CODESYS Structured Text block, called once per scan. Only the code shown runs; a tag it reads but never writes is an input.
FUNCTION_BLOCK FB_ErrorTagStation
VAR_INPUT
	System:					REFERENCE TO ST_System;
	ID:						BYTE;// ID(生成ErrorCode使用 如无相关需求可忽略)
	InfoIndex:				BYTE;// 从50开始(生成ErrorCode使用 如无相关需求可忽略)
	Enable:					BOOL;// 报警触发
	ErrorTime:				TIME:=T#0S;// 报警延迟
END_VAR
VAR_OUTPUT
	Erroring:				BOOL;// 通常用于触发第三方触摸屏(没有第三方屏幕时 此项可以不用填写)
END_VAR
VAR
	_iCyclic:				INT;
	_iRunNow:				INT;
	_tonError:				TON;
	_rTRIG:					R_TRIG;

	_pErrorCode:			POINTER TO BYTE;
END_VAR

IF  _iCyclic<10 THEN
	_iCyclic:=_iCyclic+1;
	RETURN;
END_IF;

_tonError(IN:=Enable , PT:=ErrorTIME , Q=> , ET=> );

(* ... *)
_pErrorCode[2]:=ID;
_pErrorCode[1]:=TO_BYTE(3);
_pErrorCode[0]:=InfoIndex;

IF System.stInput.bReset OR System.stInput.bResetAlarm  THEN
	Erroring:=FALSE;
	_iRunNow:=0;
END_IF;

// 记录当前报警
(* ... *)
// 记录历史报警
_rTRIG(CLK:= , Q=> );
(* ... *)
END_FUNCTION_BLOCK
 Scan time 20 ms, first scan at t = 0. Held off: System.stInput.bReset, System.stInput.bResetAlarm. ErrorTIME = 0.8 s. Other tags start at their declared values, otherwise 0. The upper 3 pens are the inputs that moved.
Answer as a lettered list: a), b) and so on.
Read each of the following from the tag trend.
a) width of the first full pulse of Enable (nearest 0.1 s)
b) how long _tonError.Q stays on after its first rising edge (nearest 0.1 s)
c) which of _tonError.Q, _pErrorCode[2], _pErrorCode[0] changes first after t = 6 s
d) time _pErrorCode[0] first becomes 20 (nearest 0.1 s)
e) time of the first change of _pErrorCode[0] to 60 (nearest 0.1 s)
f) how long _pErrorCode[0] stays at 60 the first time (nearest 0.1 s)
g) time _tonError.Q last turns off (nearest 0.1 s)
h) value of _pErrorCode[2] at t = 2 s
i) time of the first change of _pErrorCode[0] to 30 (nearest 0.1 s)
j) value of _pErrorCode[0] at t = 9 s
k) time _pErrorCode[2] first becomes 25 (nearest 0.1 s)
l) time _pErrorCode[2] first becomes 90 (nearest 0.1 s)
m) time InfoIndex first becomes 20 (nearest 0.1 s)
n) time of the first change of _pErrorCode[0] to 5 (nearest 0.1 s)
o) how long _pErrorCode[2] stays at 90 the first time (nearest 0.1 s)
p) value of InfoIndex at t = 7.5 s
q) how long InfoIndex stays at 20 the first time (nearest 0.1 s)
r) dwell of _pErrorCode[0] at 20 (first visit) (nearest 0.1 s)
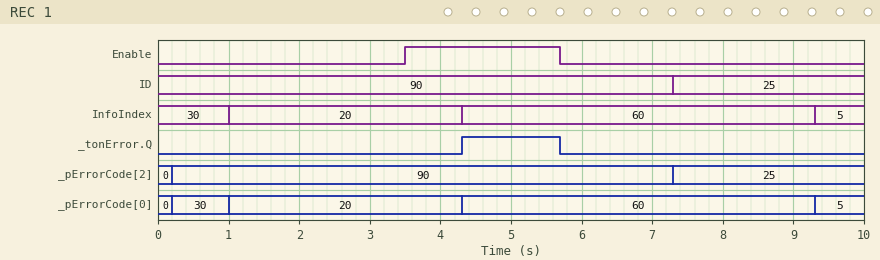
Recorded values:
a) 2.2 s
b) 1.4 s
c) _pErrorCode[2]
d) 1.0 s
e) 4.3 s
f) 5.0 s
g) 5.7 s
h) 90
i) 0.2 s
j) 60
k) 7.3 s
l) 0.2 s
m) 1.0 s
n) 9.3 s
o) 7.1 s
p) 60
q) 3.3 s
r) 3.3 s
